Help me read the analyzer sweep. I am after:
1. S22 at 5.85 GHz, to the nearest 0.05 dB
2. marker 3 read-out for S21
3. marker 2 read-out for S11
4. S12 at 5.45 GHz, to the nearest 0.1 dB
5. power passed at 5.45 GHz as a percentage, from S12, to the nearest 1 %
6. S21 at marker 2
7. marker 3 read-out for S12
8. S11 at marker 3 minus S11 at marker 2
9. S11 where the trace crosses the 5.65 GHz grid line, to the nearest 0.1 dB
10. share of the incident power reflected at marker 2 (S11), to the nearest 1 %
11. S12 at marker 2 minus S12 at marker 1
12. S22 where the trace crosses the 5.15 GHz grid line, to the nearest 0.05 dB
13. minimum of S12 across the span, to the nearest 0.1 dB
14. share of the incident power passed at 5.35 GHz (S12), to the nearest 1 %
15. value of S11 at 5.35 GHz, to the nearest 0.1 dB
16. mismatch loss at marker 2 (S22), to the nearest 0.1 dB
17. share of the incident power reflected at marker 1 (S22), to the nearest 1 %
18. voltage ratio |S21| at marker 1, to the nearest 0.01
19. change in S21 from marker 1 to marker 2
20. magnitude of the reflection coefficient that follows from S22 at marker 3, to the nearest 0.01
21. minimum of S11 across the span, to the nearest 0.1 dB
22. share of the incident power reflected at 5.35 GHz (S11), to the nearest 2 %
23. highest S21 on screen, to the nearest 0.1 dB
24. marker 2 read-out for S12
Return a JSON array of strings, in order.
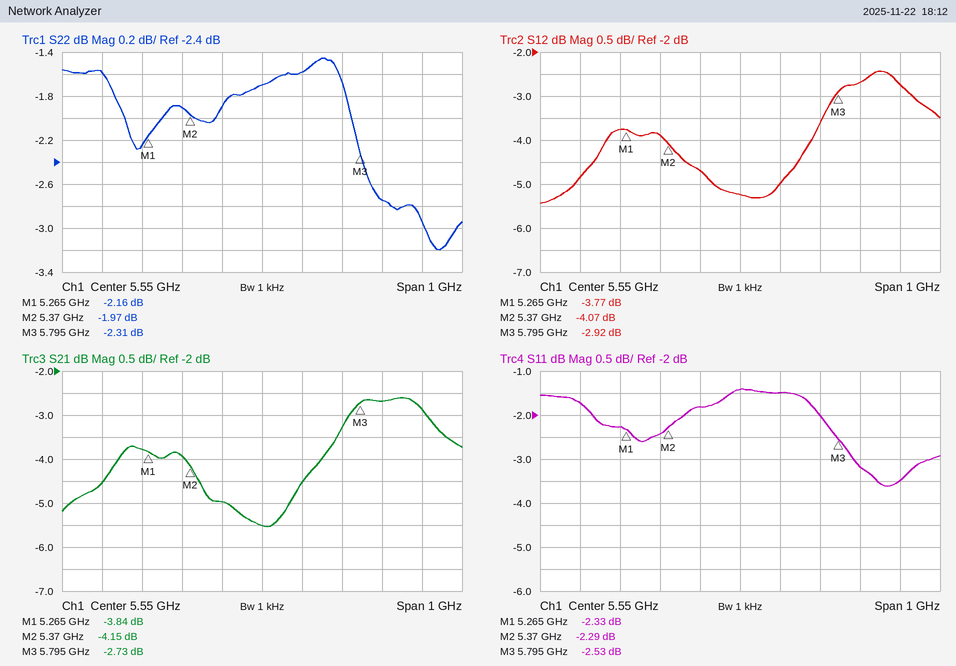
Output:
["-2.75 dB", "-2.73 dB", "-2.29 dB", "-4.7 dB", "34 %", "-4.15 dB", "-2.92 dB", "-0.24 dB", "-1.5 dB", "59 %", "-0.30 dB", "-1.60 dB", "-5.4 dB", "41 %", "-2.4 dB", "4.4 dB", "61 %", "0.64", "-0.31 dB", "0.77", "-3.6 dB", "58 %", "-2.6 dB", "-4.07 dB"]
